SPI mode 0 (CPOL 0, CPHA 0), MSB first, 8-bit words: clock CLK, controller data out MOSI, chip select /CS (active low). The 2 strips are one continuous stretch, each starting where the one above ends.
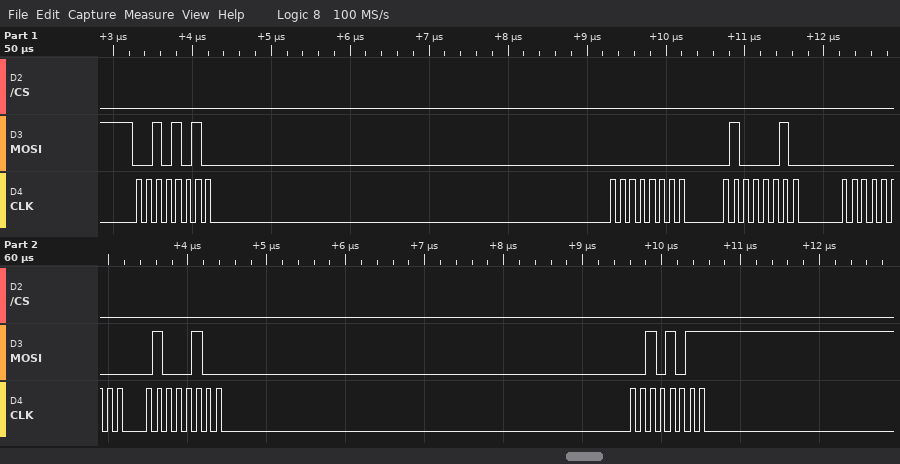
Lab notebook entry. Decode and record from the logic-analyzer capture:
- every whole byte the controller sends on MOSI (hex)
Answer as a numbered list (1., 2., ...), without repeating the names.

1. 2A 00 42 00 44 2B
